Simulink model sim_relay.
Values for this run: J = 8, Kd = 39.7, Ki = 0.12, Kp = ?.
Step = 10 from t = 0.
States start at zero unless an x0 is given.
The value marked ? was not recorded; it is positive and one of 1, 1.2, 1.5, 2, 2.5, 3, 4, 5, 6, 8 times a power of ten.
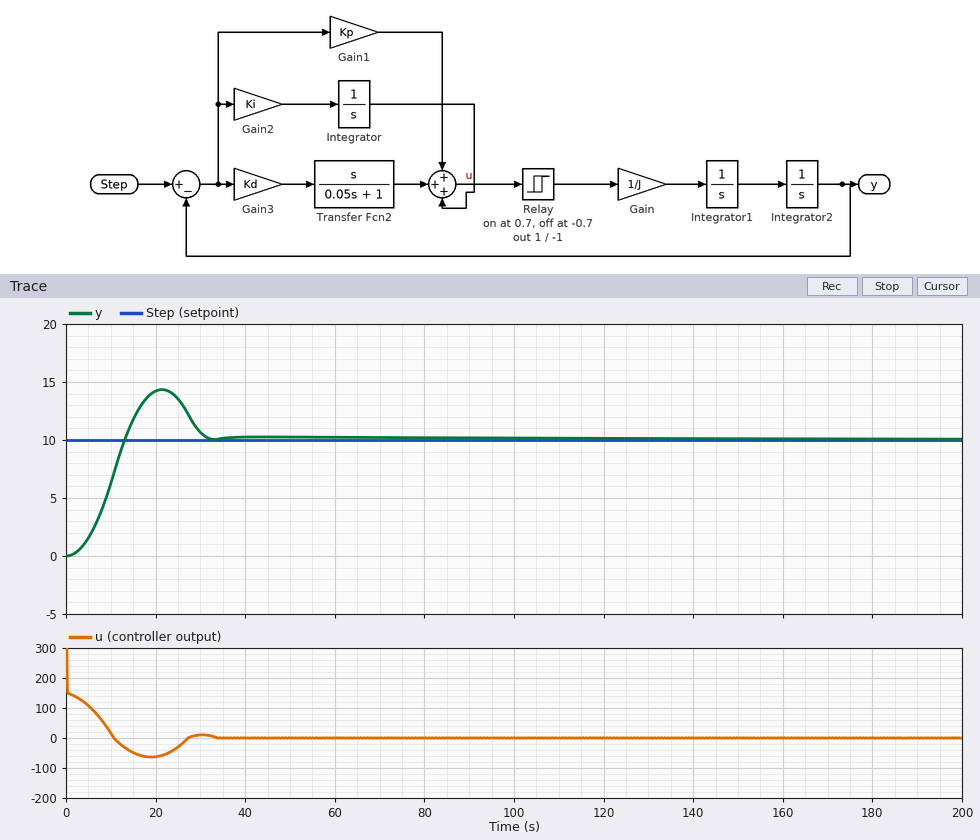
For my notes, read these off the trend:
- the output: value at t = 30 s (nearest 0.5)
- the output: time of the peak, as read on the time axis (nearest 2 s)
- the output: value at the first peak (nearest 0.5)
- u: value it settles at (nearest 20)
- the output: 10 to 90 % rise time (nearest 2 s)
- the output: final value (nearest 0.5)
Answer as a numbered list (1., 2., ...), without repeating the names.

1. 10.5
2. 22 s
3. 14.5
4. 0
5. 8 s
6. 10.0
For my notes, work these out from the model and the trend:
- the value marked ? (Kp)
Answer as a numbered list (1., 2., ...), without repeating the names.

1. 15
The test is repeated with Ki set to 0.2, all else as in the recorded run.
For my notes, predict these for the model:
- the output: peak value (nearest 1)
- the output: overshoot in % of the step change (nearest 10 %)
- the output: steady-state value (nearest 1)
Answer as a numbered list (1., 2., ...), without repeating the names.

1. 15
2. 50 %
3. 10
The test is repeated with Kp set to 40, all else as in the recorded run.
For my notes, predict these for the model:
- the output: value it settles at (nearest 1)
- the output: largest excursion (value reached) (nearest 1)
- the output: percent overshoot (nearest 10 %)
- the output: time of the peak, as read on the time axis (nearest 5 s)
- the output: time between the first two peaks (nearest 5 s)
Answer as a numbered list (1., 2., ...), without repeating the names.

1. 10
2. 18
3. 80 %
4. 25 s
5. 35 s
